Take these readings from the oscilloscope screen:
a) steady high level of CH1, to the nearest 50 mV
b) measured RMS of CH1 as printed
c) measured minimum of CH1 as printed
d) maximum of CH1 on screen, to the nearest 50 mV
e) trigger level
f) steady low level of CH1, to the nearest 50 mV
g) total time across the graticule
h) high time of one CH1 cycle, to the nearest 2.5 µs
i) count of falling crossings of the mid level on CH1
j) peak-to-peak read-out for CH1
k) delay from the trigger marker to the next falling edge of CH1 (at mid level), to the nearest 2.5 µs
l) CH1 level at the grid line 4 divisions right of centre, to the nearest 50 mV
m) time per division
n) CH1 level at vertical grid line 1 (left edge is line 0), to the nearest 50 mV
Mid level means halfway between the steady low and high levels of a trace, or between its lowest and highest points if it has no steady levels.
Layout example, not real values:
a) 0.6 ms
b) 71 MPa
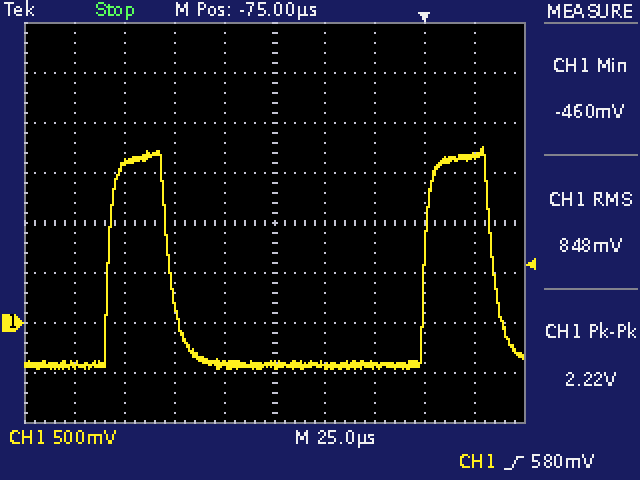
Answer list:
a) 1.65 V
b) 848 mV
c) -460 mV
d) 1.75 V
e) 580 mV
f) -400 mV
g) 250 µs
h) 32.5 µs
i) 2
j) 2.22 V
k) 35.0 µs
l) 1.65 V
m) 25 µs
n) -400 mV
